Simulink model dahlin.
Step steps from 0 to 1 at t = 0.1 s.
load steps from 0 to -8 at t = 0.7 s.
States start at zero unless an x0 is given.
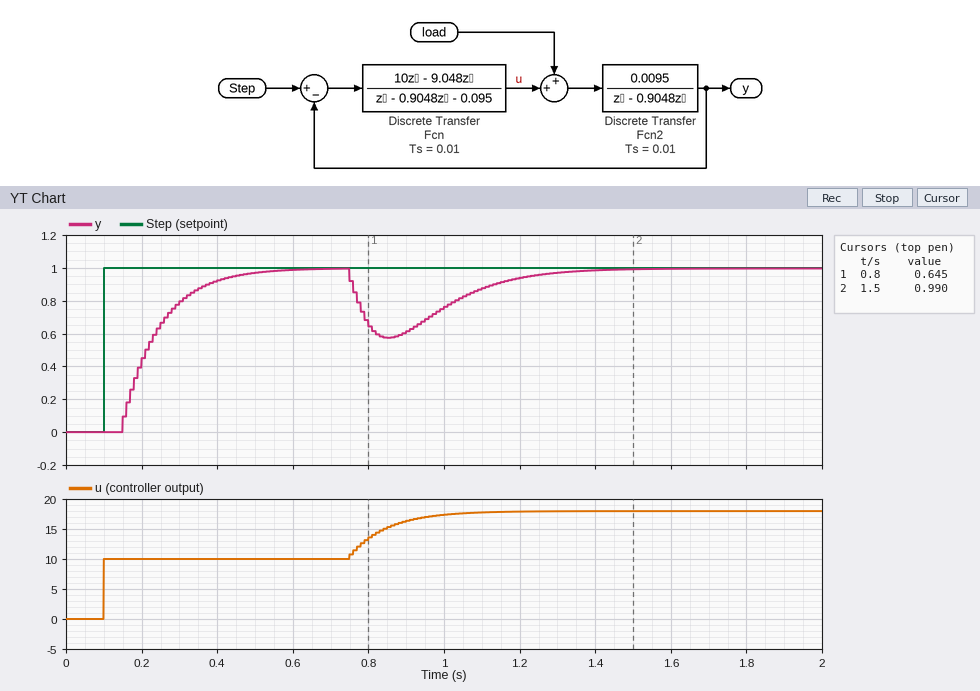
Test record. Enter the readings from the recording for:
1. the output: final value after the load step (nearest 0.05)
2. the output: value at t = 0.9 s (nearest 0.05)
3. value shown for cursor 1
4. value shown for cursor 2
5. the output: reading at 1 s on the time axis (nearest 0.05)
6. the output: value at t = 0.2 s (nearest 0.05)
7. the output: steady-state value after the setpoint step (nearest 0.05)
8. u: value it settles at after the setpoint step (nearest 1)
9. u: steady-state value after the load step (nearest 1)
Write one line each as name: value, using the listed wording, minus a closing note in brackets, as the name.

the output: final value after the load step: 1.00
the output: value at t = 0.9 s: 0.60
value shown for cursor 1: 0.645
value shown for cursor 2: 0.990
the output: reading at 1 s on the time axis: 0.75
the output: value at t = 0.2 s: 0.45
the output: steady-state value after the setpoint step: 1.00
u: value it settles at after the setpoint step: 10
u: steady-state value after the load step: 18
